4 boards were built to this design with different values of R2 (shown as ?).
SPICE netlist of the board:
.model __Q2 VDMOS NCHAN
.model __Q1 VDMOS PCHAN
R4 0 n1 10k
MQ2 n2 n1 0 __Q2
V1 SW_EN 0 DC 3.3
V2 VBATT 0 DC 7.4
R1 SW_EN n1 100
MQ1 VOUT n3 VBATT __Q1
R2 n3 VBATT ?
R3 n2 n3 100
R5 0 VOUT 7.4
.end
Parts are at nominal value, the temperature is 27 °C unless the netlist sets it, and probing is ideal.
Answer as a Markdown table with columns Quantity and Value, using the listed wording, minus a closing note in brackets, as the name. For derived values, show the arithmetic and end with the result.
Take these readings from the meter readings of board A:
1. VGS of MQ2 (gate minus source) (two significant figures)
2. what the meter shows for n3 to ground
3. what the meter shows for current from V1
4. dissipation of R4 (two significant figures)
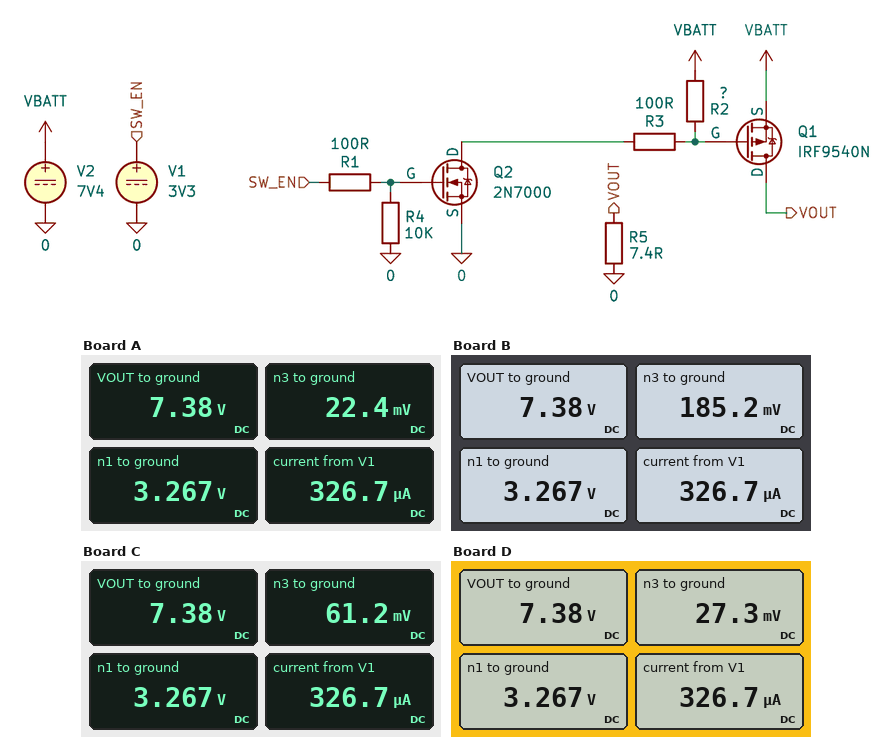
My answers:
| Quantity | Value |
|---|---|
| VGS of MQ2 (gate minus source) | 3.267 V = 3.3 V |
| what the meter shows for n3 to ground | 22.4 mV |
| what the meter shows for current from V1 | 326.7 µA |
| dissipation of R4 | (3.267 V)^2 / 10 kΩ = 1.1 mW |
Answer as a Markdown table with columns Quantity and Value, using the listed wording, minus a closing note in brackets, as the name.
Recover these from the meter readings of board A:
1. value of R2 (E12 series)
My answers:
| Quantity | Value |
|---|---|
| value of R2 | 33 kΩ |
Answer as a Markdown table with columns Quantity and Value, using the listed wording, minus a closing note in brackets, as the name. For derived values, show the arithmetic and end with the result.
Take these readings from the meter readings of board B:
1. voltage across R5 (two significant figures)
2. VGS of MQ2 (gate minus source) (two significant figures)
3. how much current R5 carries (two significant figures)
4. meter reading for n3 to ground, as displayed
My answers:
| Quantity | Value |
|---|---|
| voltage across R5 | 7.38 V = 7.4 V |
| VGS of MQ2 (gate minus source) | 3.267 V = 3.3 V |
| how much current R5 carries | (7.38 V) / 7.4 Ω = 1.0 A |
| meter reading for n3 to ground, as displayed | 185.2 mV |
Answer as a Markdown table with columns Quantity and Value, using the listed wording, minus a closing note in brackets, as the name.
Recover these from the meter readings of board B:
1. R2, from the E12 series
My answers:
| Quantity | Value |
|---|---|
| R2, from the E12 series | 3.9 kΩ |
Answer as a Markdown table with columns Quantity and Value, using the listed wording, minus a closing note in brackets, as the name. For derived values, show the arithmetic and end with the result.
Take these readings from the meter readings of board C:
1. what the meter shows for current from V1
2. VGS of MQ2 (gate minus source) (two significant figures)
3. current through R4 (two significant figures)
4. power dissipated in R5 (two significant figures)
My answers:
| Quantity | Value |
|---|---|
| what the meter shows for current from V1 | 326.7 µA |
| VGS of MQ2 (gate minus source) | 3.267 V = 3.3 V |
| current through R4 | (3.267 V) / 10 kΩ = 330 µA |
| power dissipated in R5 | (7.38 V)^2 / 7.4 Ω = 7.4 W |
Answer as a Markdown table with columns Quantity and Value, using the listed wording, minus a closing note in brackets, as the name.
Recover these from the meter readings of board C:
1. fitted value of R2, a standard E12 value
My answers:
| Quantity | Value |
|---|---|
| fitted value of R2, a standard E12 value | 12 kΩ |
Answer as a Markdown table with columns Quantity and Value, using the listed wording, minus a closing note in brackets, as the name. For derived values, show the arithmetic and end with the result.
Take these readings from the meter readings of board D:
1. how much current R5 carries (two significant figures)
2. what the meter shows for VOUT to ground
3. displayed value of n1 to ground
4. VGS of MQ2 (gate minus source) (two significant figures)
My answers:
| Quantity | Value |
|---|---|
| how much current R5 carries | (7.38 V) / 7.4 Ω = 1.0 A |
| what the meter shows for VOUT to ground | 7.38 V |
| displayed value of n1 to ground | 3.267 V |
| VGS of MQ2 (gate minus source) | 3.267 V = 3.3 V |
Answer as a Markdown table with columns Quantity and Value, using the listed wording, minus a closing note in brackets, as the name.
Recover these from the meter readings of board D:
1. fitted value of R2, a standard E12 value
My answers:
| Quantity | Value |
|---|---|
| fitted value of R2, a standard E12 value | 27 kΩ |
